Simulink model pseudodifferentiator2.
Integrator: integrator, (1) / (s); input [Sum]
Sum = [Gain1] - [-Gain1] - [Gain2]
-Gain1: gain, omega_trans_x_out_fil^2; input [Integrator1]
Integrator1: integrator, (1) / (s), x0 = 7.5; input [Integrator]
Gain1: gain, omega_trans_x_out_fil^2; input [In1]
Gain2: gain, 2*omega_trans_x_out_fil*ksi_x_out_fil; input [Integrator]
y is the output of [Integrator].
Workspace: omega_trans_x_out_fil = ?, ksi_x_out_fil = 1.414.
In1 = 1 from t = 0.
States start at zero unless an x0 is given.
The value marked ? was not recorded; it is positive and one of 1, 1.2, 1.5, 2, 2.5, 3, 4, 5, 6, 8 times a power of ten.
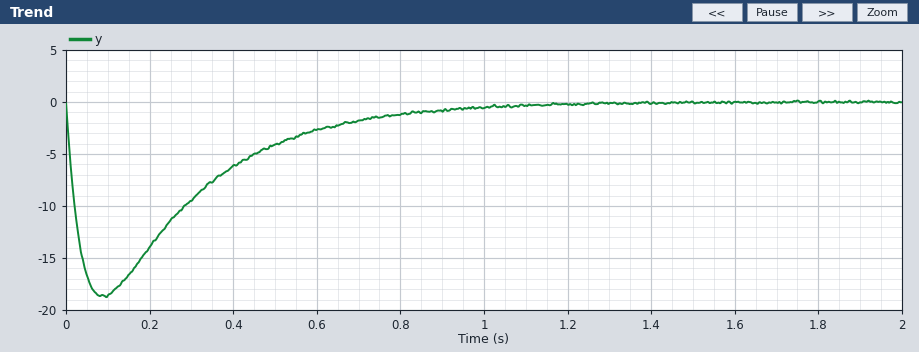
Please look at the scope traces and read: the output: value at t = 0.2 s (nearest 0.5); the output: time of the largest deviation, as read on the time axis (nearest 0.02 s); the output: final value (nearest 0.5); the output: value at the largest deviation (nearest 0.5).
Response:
-14.0
0.08 s
0.0
-18.5
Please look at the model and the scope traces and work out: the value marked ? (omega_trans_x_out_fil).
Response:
10
